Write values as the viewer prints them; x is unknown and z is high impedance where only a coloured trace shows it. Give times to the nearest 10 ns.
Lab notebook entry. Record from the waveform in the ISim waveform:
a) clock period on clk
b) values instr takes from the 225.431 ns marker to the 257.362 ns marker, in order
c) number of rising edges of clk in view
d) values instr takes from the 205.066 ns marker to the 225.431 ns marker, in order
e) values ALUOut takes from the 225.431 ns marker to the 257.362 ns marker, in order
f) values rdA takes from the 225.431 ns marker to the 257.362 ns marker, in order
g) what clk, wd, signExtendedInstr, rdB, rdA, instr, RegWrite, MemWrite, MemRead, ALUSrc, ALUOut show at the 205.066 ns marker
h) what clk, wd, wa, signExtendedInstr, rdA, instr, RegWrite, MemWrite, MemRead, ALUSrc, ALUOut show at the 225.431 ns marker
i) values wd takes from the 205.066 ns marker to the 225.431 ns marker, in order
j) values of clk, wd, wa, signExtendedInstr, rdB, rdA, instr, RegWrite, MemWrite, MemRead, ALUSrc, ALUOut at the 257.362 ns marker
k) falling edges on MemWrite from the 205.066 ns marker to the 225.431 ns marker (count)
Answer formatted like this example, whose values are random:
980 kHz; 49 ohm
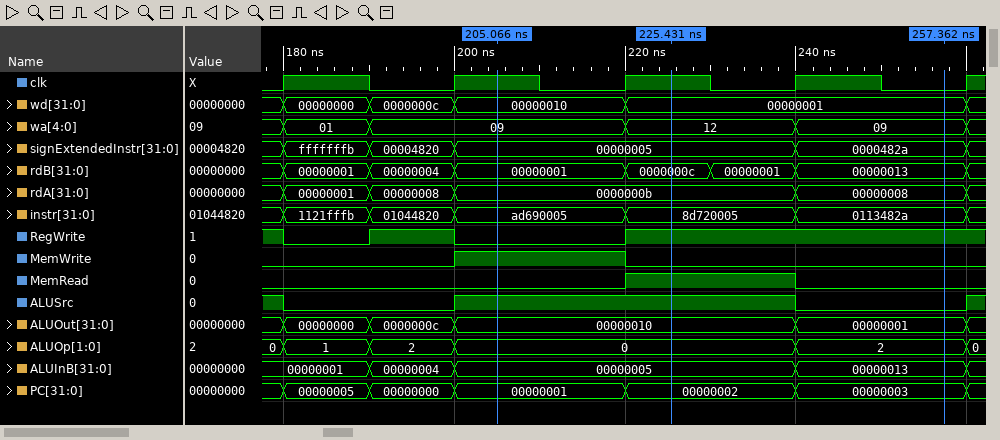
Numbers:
20 ns; 8d720005, 0113482a; 5; ad690005, 8d720005; 00000010, 00000001; 0000000b, 00000008; clk=1, wd=00000010, signExtendedInstr=00000005, rdB=00000001, rdA=0000000b, instr=ad690005, RegWrite=0, MemWrite=1, MemRead=0, ALUSrc=1, ALUOut=00000010; clk=1, wd=00000001, wa=12, signExtendedInstr=00000005, rdA=0000000b, instr=8d720005, RegWrite=1, MemWrite=0, MemRead=1, ALUSrc=1, ALUOut=00000010; 00000010, 00000001; clk=0, wd=00000001, wa=09, signExtendedInstr=0000482a, rdB=00000013, rdA=00000008, instr=0113482a, RegWrite=1, MemWrite=0, MemRead=0, ALUSrc=0, ALUOut=00000001; 1
